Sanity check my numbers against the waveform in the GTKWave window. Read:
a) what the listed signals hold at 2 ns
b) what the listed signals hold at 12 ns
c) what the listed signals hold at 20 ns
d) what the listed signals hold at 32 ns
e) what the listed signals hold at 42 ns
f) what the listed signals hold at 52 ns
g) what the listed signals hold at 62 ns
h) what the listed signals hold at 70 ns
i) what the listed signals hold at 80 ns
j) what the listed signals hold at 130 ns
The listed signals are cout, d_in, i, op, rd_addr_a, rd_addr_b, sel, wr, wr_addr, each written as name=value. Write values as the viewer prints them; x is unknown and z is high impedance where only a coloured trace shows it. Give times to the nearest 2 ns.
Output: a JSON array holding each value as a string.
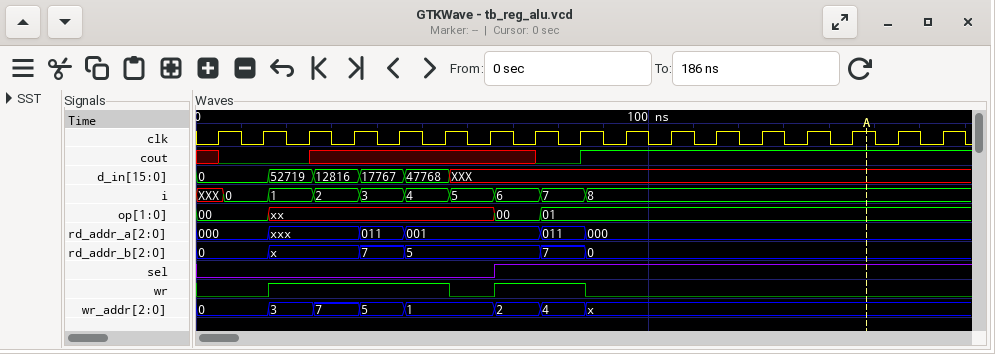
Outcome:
["cout=x, d_in=0, i=XXX, op=00, rd_addr_a=000, rd_addr_b=0, sel=0, wr=0, wr_addr=0", "cout=0, d_in=0, i=0, op=00, rd_addr_a=000, rd_addr_b=0, sel=0, wr=0, wr_addr=0", "cout=0, d_in=52719, i=1, op=xx, rd_addr_a=xxx, rd_addr_b=x, sel=0, wr=1, wr_addr=3", "cout=x, d_in=12816, i=2, op=xx, rd_addr_a=xxx, rd_addr_b=x, sel=0, wr=1, wr_addr=7", "cout=x, d_in=17767, i=3, op=xx, rd_addr_a=011, rd_addr_b=7, sel=0, wr=1, wr_addr=5", "cout=x, d_in=47768, i=4, op=xx, rd_addr_a=001, rd_addr_b=5, sel=0, wr=1, wr_addr=1", "cout=x, d_in=XXX, i=5, op=xx, rd_addr_a=001, rd_addr_b=5, sel=0, wr=0, wr_addr=1", "cout=x, d_in=XXX, i=6, op=00, rd_addr_a=001, rd_addr_b=5, sel=1, wr=1, wr_addr=2", "cout=0, d_in=XXX, i=7, op=01, rd_addr_a=011, rd_addr_b=7, sel=1, wr=1, wr_addr=4", "cout=1, d_in=XXX, i=8, op=01, rd_addr_a=000, rd_addr_b=0, sel=1, wr=0, wr_addr=x"]
